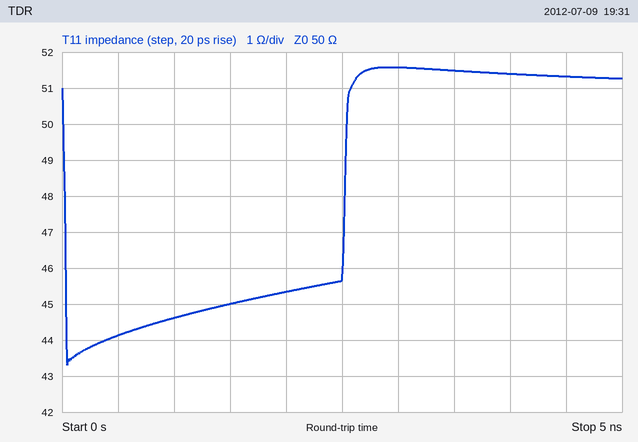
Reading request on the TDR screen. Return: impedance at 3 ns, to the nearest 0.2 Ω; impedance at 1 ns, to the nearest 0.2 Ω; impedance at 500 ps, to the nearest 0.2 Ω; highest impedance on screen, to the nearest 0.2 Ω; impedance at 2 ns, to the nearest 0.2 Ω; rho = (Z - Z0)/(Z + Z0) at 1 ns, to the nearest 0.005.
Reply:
51.6 Ω
44.6 Ω
44.2 Ω
51.6 Ω
45.4 Ω
-0.055
